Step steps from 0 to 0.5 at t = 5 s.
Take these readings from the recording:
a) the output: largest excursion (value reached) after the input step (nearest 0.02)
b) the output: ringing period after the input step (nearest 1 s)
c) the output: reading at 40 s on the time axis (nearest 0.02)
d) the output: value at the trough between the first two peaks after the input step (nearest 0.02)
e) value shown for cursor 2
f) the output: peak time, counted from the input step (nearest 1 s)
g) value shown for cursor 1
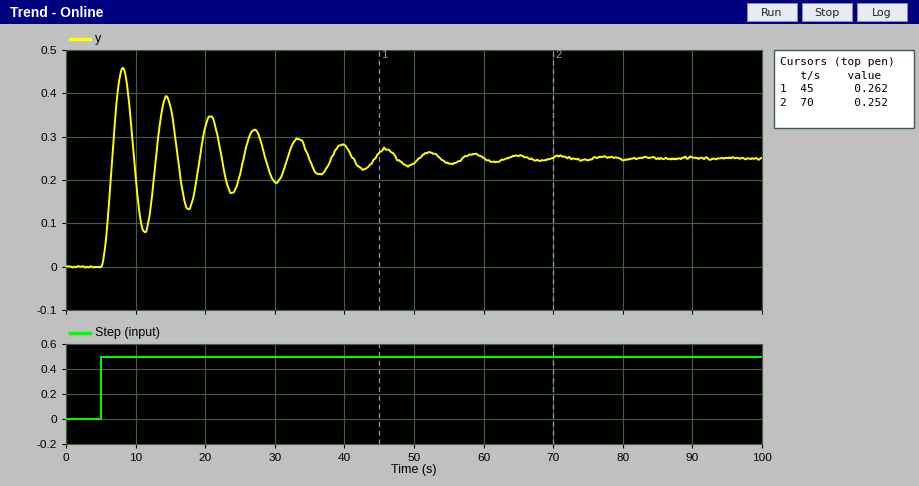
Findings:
0.46
6 s
0.28
0.08
0.252
3 s
0.262
